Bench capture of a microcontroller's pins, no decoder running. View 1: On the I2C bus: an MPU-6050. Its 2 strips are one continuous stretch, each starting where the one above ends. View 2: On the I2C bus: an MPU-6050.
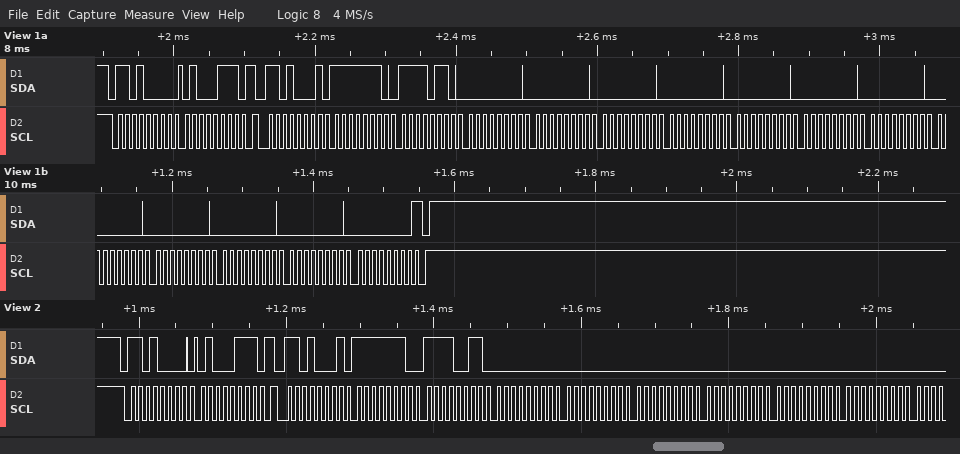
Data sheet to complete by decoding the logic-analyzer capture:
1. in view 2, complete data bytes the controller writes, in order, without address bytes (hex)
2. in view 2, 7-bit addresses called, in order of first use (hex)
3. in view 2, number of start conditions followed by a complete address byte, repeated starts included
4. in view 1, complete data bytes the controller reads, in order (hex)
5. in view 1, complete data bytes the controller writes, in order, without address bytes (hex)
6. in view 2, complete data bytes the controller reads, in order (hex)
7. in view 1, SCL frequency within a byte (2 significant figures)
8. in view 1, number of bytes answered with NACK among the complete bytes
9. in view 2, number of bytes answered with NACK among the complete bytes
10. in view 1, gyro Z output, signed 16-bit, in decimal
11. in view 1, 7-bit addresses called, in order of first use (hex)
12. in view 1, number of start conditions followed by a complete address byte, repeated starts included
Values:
47
0x68
2
FE F6 00 00 00 00 00 00 00 00 00 00 00 00
47
FE F3 00 00 00 00 00 00
100 kHz
1
0
-266
0x68
2
